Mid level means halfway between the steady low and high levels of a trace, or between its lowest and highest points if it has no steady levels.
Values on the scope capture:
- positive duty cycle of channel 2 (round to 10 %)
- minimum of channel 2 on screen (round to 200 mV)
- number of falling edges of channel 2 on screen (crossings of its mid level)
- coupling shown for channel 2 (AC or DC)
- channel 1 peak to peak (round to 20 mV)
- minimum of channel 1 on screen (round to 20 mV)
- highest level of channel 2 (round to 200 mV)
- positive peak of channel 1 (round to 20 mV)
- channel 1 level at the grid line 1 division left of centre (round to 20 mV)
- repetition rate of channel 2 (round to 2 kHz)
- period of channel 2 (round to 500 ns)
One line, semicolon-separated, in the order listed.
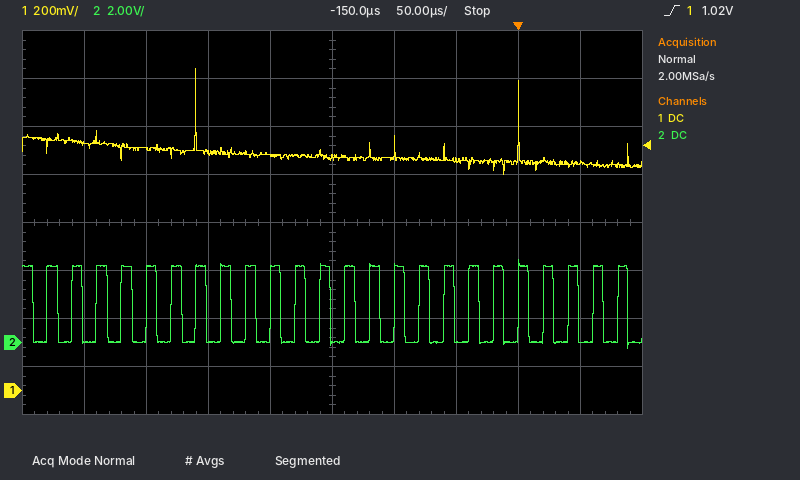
40 %; -200 mV; 25; DC; 440 mV; 900 mV; 3.4 V; 1.34 V; 980 mV; 50 kHz; 20.0 µs
